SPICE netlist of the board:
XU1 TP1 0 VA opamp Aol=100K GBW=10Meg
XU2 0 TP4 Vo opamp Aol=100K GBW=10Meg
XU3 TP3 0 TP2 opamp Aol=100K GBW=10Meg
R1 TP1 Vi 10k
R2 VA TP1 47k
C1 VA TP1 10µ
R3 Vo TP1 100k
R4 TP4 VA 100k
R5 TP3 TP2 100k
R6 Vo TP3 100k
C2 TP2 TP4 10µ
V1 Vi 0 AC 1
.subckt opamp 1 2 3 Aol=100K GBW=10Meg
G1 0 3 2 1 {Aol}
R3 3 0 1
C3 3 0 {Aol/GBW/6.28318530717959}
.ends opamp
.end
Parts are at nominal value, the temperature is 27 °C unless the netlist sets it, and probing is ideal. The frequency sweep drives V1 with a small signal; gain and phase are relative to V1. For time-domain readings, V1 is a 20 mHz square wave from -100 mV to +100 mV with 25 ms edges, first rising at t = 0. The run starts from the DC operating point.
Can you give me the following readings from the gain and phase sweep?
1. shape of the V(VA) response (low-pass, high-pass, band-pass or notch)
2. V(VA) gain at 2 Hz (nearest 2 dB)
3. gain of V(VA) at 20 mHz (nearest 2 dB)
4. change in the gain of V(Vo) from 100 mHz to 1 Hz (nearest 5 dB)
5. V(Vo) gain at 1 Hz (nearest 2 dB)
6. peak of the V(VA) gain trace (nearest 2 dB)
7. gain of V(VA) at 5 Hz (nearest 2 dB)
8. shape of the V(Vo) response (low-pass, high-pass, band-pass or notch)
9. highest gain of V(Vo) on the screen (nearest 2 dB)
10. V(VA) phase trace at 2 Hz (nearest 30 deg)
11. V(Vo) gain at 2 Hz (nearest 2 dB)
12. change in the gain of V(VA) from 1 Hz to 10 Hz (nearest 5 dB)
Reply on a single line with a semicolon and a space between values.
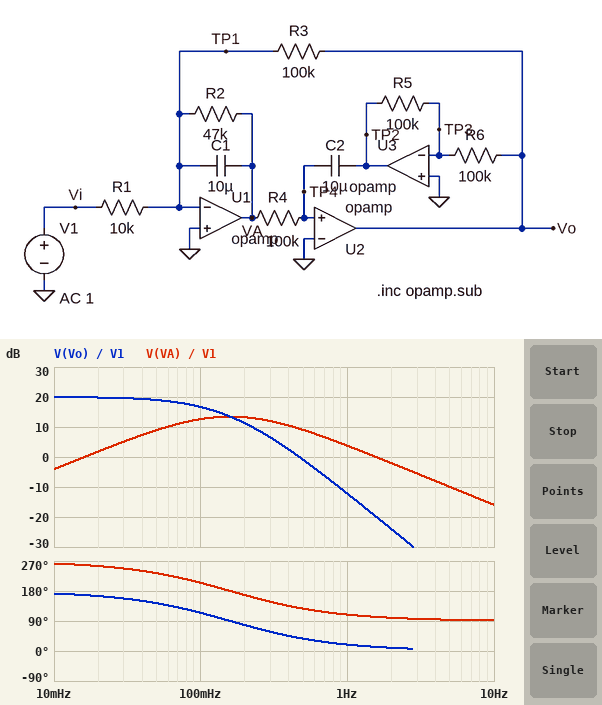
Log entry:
band-pass; -2 dB; 2 dB; -30 dB; -12 dB; 14 dB; -10 dB; low-pass; 20 dB; 90 deg; -24 dB; -20 dB
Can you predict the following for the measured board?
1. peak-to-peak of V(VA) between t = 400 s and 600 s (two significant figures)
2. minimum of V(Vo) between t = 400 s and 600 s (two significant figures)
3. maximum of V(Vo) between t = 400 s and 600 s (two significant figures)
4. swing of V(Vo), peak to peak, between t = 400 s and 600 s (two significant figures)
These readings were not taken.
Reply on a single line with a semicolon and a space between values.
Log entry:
1.4 V; -1.0 V; 1.0 V; 2.0 V
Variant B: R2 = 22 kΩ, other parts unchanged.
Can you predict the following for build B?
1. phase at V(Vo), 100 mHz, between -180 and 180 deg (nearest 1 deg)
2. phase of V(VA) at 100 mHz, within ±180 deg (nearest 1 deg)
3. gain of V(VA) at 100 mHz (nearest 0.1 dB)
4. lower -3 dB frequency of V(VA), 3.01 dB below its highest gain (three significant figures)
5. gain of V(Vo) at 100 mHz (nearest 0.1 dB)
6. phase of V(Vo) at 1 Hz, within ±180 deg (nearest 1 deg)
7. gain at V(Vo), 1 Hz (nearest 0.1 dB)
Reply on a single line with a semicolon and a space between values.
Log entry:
102 deg; -168 deg; 6.7 dB; 33.5 mHz; 10.7 dB; 37 deg; -13.6 dB
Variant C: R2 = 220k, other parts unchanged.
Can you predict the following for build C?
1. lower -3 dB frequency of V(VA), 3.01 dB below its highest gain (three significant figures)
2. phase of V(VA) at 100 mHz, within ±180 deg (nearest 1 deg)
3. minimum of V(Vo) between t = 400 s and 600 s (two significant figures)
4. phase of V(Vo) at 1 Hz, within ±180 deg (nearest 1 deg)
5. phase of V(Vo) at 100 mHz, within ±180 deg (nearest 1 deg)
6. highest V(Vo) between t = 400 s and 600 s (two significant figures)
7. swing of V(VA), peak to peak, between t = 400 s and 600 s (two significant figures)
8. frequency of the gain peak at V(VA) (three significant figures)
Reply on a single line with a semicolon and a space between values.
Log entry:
127 mHz; -115 deg; -2.0 V; 4 deg; 155 deg; 2.0 V; 2.9 V; 159 mHz
